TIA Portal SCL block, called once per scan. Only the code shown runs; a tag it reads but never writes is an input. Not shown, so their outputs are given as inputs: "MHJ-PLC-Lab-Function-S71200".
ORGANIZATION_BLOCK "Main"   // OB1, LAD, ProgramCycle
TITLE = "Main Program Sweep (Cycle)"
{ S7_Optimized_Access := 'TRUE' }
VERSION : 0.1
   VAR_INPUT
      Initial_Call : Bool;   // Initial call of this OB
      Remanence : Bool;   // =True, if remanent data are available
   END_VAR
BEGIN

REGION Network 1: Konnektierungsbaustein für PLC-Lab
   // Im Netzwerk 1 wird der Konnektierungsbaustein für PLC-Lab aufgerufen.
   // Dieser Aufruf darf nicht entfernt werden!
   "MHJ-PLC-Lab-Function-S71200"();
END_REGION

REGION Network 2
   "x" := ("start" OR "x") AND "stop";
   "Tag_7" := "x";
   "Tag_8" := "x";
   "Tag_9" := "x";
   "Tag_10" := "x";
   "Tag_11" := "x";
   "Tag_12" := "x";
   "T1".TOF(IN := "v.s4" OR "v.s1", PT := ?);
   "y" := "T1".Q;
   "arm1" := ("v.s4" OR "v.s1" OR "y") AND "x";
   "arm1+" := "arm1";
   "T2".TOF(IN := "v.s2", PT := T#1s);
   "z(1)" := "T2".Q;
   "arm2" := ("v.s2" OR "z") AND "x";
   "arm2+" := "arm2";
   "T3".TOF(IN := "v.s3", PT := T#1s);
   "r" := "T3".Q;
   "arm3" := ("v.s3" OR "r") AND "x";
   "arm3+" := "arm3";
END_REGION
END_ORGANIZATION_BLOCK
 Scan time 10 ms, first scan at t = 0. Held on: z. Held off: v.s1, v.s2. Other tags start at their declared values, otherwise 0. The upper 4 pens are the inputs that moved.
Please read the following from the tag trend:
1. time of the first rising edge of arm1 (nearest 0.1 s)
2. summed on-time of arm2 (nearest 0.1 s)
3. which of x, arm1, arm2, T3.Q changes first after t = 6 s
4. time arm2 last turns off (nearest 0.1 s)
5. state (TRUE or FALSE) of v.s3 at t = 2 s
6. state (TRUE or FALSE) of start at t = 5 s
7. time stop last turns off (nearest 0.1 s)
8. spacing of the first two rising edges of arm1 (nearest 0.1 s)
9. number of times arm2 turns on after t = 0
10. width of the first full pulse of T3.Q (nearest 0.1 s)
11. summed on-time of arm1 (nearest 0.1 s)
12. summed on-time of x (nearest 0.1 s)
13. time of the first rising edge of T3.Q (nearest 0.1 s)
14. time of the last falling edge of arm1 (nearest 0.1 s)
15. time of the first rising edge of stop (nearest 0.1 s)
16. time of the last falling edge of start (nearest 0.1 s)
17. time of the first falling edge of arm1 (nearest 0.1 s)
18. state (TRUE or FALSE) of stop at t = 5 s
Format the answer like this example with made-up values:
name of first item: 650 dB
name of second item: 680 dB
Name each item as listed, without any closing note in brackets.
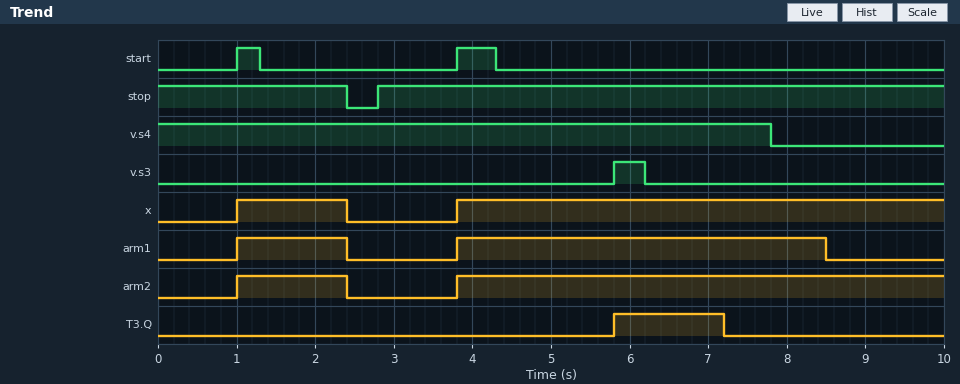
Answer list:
time of the first rising edge of arm1: 1.0 s
summed on-time of arm2: 7.6 s
which of x, arm1, arm2, T3.Q changes first after t = 6 s: T3.Q
time arm2 last turns off: 2.4 s
state (TRUE or FALSE) of v.s3 at t = 2 s: FALSE
state (TRUE or FALSE) of start at t = 5 s: FALSE
time stop last turns off: 2.4 s
spacing of the first two rising edges of arm1: 2.8 s
number of times arm2 turns on after t = 0: 2
width of the first full pulse of T3.Q: 1.4 s
summed on-time of arm1: 6.1 s
summed on-time of x: 7.6 s
time of the first rising edge of T3.Q: 5.8 s
time of the last falling edge of arm1: 8.5 s
time of the first rising edge of stop: 2.8 s
time of the last falling edge of start: 4.3 s
time of the first falling edge of arm1: 2.4 s
state (TRUE or FALSE) of stop at t = 5 s: TRUE
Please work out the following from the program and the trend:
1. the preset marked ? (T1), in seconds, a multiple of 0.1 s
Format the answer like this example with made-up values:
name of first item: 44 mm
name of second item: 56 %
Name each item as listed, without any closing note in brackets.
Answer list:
the preset marked ? (T1), in seconds, a multiple of 0.1 s: 0.7 s
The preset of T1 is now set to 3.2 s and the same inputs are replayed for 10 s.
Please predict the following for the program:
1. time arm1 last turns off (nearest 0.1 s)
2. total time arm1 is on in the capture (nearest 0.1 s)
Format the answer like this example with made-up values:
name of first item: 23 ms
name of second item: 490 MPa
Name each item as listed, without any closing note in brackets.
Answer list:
time arm1 last turns off: 2.4 s
total time arm1 is on in the capture: 7.6 s
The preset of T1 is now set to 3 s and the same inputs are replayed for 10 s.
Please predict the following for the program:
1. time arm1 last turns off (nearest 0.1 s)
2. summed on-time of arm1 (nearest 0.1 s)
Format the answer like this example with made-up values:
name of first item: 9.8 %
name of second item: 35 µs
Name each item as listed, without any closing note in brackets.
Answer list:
time arm1 last turns off: 2.4 s
summed on-time of arm1: 7.6 s
